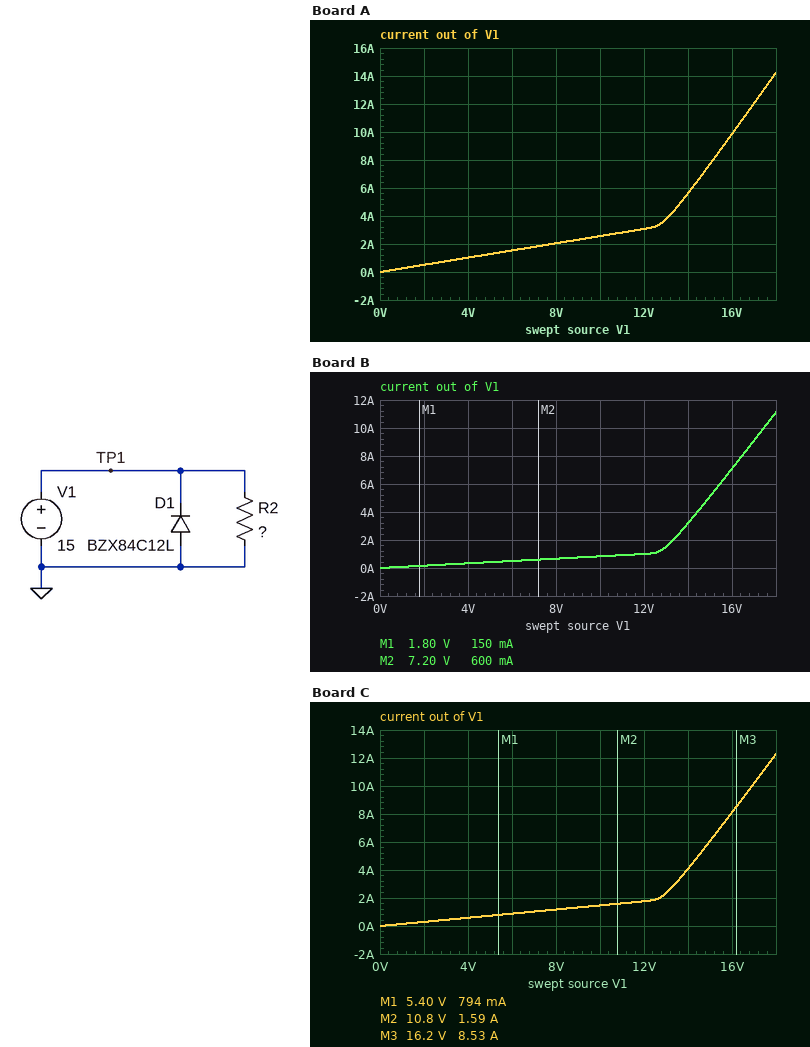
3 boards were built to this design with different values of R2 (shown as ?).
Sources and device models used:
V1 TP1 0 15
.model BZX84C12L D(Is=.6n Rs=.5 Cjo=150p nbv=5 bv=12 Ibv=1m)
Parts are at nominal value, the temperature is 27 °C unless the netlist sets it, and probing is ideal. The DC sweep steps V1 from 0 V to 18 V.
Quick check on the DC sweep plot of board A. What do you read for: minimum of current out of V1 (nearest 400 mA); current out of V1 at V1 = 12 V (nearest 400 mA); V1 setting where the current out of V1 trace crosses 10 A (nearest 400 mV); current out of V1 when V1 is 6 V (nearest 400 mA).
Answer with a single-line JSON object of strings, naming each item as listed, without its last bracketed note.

{"minimum of current out of V1": "0 A", "current out of V1 at V1 = 12 V": "3.2 A", "V1 setting where the current out of V1 trace crosses 10 A": "16.0 V", "current out of V1 when V1 is 6 V": "1.6 A"}
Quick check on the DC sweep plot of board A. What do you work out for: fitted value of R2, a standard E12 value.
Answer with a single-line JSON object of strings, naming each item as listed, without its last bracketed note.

{"fitted value of R2, a standard E12 value": "3.9 Ω"}
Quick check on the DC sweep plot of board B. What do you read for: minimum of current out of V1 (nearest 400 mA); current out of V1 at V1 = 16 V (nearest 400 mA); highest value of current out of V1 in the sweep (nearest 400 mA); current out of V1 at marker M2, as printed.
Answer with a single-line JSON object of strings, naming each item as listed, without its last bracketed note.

{"minimum of current out of V1": "0 A", "current out of V1 at V1 = 16 V": "7.2 A", "highest value of current out of V1 in the sweep": "11.2 A", "current out of V1 at marker M2, as printed": "600 mA"}
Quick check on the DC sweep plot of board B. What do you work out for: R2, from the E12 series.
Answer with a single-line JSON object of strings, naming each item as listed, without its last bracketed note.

{"R2, from the E12 series": "12 Ω"}
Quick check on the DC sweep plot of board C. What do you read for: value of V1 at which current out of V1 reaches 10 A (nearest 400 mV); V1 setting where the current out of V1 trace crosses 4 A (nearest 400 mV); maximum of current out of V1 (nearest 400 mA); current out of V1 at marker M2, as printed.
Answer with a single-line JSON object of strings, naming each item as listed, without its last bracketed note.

{"value of V1 at which current out of V1 reaches 10 A": "16.8 V", "V1 setting where the current out of V1 trace crosses 4 A": "14.0 V", "maximum of current out of V1": "12.4 A", "current out of V1 at marker M2, as printed": "1.59 A"}
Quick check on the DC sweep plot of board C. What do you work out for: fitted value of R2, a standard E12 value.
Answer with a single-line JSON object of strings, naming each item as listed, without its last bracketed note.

{"fitted value of R2, a standard E12 value": "6.8 Ω"}
